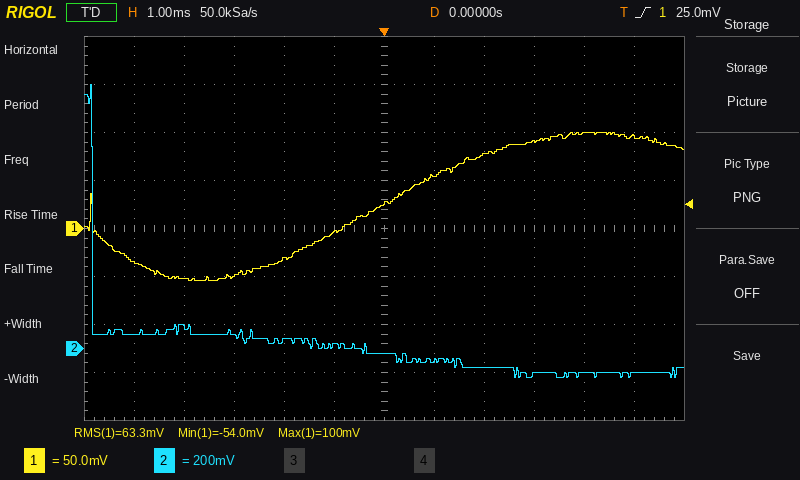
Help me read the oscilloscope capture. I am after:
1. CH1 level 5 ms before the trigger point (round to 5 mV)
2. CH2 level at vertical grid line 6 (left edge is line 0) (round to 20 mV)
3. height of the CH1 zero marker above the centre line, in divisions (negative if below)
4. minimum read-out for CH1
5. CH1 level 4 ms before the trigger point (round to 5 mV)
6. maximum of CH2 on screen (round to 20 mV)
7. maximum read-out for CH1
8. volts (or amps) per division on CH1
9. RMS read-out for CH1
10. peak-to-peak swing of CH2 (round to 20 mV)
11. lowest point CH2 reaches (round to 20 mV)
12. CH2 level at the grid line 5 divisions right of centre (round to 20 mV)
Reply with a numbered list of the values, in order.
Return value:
1. -35 mV
2. -20 mV
3. 0.0 div
4. -54.0 mV
5. -50 mV
6. 1.10 V
7. 100 mV
8. 50 mV
9. 63.3 mV
10. 1.22 V
11. -120 mV
12. -100 mV
